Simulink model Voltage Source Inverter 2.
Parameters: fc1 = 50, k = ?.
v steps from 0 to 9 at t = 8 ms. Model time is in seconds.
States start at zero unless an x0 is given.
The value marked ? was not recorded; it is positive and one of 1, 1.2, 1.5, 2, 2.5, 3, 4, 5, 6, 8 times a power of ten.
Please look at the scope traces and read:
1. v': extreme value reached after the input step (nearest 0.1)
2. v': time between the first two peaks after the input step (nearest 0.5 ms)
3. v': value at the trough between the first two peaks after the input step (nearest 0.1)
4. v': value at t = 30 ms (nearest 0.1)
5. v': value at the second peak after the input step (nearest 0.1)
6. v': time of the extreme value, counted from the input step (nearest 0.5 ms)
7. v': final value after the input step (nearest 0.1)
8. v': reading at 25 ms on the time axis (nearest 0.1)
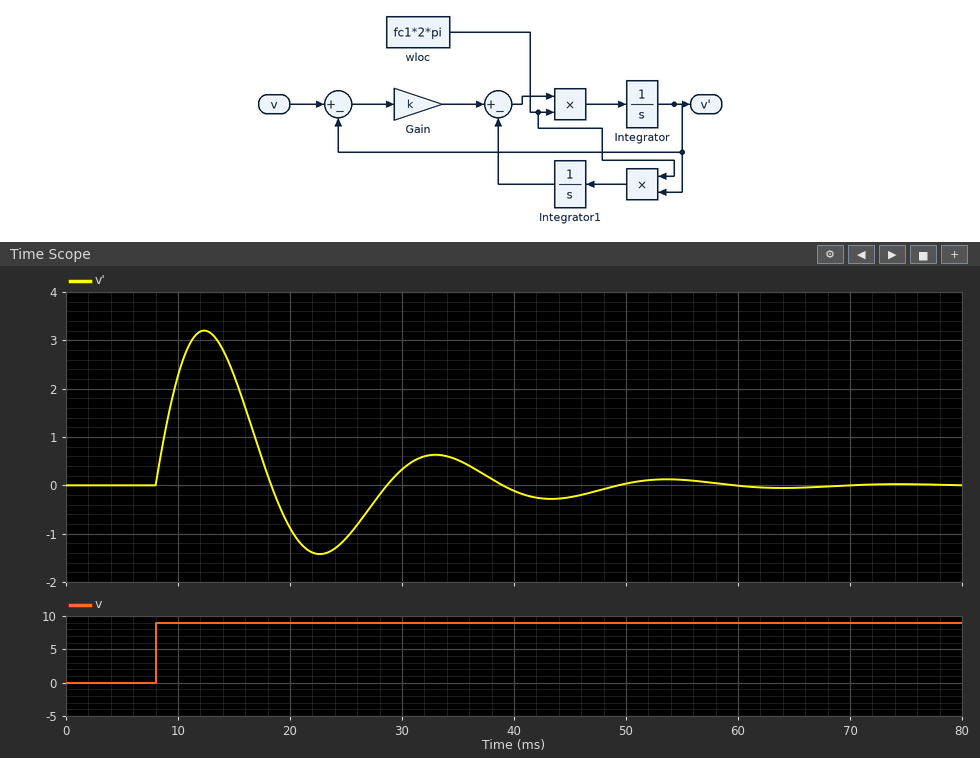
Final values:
3.2
20.5 ms
-1.4
0.3
0.6
4.5 ms
0.0
-1.1
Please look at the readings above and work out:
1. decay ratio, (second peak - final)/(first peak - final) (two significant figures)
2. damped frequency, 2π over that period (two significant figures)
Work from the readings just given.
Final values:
0.19
0.31 rad/ms
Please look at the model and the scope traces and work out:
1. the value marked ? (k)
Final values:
0.5
